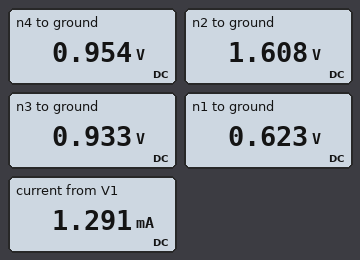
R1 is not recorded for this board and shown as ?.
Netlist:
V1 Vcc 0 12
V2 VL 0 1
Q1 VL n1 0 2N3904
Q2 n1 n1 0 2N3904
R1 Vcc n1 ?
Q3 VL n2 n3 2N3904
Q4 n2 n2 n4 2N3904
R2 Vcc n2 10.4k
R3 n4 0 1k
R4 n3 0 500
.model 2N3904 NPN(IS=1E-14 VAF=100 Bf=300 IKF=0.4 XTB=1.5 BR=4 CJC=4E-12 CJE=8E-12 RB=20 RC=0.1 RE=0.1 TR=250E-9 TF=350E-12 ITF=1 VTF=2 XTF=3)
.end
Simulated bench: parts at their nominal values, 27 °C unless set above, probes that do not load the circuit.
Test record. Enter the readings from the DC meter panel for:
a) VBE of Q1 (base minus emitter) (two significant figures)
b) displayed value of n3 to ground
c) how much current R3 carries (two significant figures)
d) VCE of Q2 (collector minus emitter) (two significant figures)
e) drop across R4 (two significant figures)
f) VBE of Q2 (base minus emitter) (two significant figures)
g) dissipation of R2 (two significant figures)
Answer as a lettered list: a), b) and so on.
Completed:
a) 620 mV
b) 0.933 V
c) 950 µA
d) 620 mV
e) 930 mV
f) 620 mV
g) 10 mW
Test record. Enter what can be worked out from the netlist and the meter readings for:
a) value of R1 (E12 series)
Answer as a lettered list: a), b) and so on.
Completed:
a) 39 kΩ
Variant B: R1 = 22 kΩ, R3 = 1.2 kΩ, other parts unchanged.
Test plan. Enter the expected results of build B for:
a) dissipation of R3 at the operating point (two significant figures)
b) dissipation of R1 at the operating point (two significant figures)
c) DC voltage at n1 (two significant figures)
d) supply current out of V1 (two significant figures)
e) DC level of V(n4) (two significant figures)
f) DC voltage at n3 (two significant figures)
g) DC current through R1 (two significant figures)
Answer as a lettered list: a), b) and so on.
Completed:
a) 830 µW
b) 5.9 mW
c) 640 mV
d) 1.5 mA
e) 1.0 V
f) 960 mV
g) 520 µA
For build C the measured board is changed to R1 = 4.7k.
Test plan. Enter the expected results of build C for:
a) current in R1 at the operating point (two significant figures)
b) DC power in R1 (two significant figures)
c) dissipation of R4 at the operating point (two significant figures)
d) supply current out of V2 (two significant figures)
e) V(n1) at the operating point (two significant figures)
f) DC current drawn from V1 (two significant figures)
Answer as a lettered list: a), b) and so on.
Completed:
a) 2.4 mA
b) 27 mW
c) 1.7 mW
d) 4.2 mA
e) 680 mV
f) 3.4 mA
